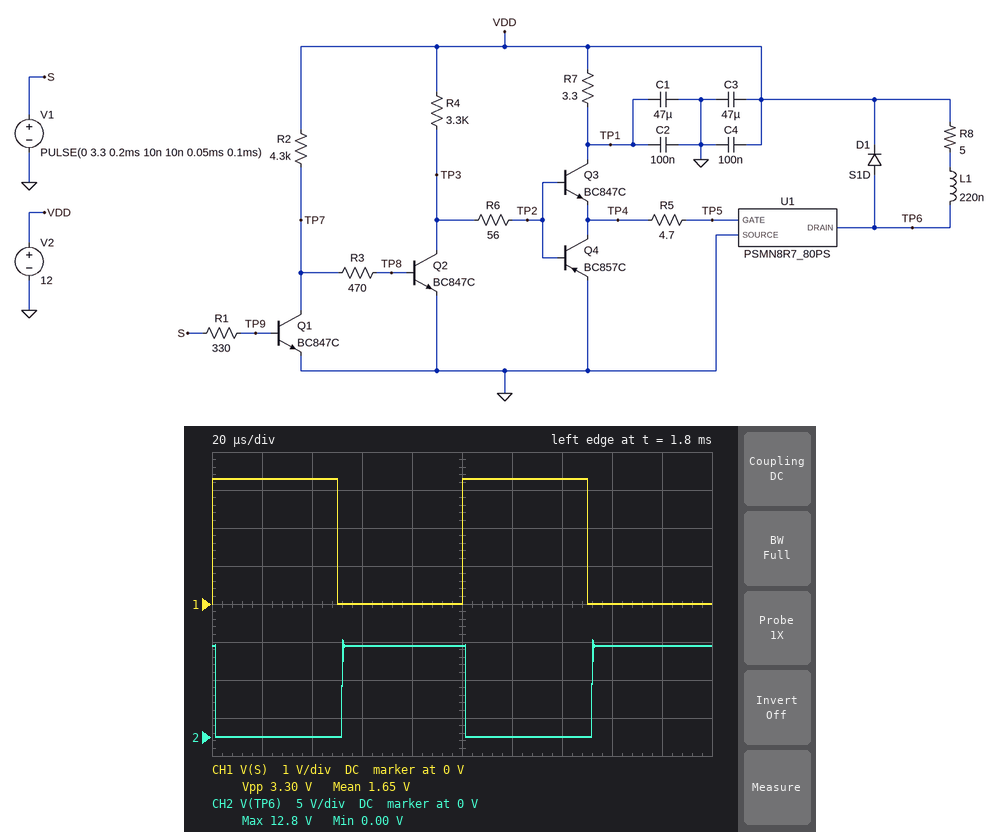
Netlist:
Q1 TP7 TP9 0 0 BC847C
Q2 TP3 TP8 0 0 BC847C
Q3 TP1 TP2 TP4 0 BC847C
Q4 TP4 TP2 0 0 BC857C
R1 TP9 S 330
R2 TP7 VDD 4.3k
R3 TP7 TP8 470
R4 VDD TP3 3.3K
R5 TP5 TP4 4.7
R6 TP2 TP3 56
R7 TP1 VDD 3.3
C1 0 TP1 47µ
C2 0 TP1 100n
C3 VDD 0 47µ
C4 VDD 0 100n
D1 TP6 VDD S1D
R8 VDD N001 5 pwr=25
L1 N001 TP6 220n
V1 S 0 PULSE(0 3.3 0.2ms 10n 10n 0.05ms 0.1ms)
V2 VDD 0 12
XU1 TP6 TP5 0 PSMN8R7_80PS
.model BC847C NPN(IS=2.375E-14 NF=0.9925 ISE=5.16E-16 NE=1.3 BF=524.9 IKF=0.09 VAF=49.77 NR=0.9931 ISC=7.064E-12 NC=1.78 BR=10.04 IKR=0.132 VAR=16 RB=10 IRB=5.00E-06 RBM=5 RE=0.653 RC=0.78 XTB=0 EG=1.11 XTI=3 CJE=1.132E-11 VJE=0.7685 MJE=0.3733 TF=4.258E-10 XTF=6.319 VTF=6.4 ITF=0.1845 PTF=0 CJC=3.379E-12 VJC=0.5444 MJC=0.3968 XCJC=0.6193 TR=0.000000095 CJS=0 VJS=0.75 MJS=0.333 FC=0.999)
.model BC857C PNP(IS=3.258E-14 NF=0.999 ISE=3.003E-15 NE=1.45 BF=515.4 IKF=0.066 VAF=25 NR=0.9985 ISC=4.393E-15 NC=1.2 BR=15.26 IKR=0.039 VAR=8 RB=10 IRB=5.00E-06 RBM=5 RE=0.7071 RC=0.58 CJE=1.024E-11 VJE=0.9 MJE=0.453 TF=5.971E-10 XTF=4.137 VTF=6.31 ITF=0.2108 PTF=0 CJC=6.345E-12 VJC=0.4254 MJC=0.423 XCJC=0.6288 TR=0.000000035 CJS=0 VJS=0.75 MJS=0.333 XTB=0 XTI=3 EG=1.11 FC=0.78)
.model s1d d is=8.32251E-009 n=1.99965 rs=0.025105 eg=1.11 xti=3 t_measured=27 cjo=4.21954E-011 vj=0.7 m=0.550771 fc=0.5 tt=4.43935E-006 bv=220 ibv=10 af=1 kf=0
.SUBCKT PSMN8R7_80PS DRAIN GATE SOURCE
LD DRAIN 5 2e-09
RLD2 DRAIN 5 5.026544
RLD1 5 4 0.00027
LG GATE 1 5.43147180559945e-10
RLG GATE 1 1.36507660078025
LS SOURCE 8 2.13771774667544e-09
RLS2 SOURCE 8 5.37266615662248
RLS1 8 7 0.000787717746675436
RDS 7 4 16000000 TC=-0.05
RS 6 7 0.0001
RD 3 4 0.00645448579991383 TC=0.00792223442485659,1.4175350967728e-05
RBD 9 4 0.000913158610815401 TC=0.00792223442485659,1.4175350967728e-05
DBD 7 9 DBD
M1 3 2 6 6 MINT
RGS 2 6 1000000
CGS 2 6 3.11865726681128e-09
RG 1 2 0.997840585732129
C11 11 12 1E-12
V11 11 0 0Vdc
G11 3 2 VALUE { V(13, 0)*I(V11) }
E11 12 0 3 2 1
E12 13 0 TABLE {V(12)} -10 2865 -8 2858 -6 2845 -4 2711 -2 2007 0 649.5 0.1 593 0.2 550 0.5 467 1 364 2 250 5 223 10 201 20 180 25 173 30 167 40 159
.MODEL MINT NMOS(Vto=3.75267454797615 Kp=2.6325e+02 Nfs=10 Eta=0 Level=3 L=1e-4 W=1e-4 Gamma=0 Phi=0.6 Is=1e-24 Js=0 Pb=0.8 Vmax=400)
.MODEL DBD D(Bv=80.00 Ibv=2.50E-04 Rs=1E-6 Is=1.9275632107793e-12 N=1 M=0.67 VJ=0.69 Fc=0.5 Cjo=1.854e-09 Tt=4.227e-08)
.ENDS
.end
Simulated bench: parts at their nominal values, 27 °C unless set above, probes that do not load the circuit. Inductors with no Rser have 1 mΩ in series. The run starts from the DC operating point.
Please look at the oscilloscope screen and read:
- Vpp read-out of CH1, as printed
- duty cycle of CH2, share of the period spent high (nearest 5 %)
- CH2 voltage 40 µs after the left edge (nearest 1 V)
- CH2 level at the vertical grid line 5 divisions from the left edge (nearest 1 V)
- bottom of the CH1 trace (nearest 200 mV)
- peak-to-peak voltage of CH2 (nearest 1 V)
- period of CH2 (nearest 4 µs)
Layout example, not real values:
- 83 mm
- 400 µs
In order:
- 3.30 V
- 50 %
- 0 V
- 12 V
- 0 V
- 13 V
- 100 µs
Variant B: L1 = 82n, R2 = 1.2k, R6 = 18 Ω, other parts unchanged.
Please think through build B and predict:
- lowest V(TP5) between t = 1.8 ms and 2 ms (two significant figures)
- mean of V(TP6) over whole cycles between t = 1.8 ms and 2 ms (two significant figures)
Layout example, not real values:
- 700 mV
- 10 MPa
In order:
- -94 mV
- 6.0 V
